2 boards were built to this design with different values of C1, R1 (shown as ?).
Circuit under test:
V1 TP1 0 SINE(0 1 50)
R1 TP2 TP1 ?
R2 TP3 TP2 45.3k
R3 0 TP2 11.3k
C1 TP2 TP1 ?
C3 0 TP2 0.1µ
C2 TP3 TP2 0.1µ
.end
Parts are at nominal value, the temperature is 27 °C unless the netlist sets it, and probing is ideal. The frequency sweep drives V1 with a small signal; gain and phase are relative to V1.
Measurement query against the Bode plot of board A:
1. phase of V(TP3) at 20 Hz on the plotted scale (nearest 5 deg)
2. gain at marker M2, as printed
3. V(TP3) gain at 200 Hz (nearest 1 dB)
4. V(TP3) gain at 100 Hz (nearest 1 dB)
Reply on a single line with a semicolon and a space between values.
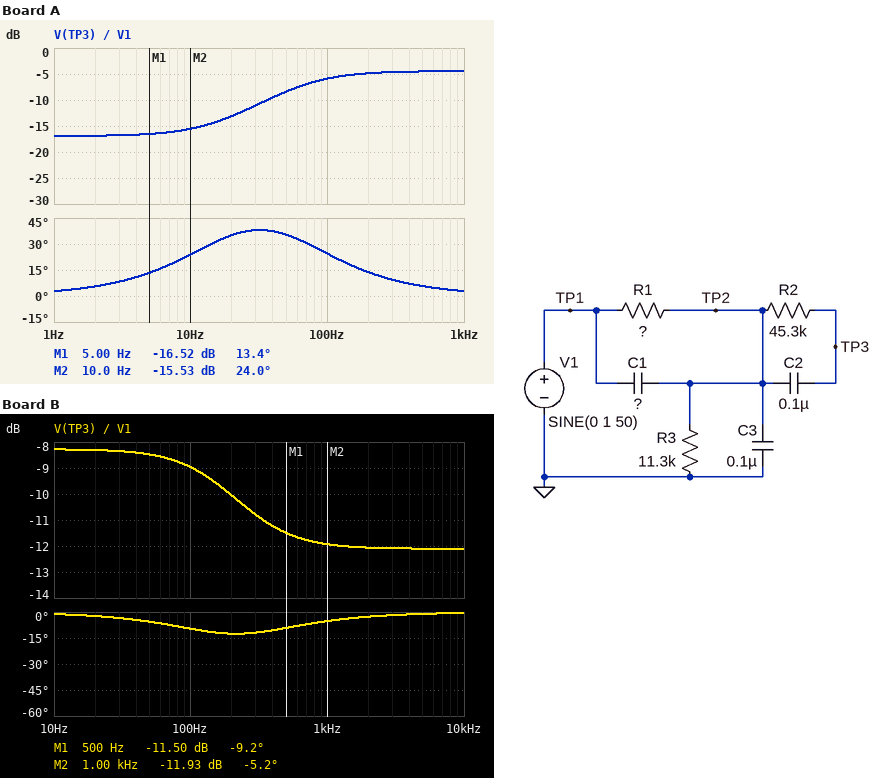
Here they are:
35 deg; -15.53 dB; -5 dB; -6 dB
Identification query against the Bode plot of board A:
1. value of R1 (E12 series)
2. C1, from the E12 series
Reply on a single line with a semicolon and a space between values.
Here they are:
68 kΩ; 150 nF
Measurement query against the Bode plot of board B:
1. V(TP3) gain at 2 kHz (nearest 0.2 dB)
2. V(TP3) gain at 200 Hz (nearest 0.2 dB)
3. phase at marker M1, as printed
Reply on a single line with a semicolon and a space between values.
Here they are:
-12.0 dB; -10.0 dB; -9.2 deg
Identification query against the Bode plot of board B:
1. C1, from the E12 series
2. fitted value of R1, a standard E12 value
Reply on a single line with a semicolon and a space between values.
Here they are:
33 nF; 18 kΩ
